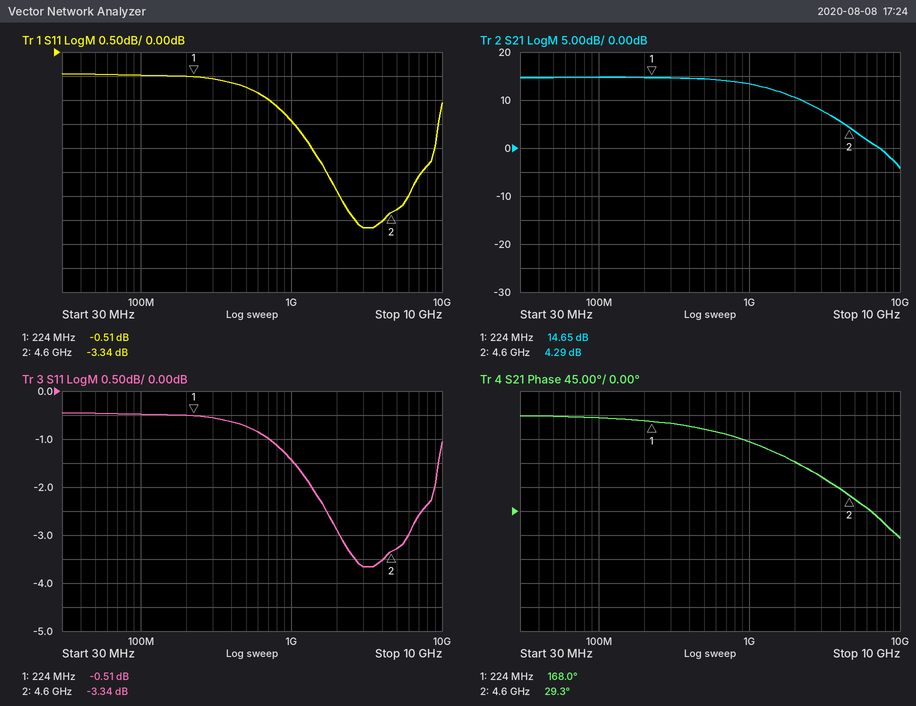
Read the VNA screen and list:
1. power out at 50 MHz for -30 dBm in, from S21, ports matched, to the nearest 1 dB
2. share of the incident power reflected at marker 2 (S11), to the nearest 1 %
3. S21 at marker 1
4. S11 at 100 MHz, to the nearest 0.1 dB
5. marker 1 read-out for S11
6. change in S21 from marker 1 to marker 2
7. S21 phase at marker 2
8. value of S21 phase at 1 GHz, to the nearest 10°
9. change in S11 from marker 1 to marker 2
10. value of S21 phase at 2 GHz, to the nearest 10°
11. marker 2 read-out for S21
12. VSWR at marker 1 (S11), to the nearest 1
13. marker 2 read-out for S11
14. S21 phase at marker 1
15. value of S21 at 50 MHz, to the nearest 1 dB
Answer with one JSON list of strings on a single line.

["-15 dBm", "46 %", "14.65 dB", "-0.5 dB", "-0.51 dB", "-10.36 dB", "29.3°", "130°", "-2.83 dB", "90°", "4.29 dB", "34", "-3.34 dB", "168.0°", "15 dB"]
